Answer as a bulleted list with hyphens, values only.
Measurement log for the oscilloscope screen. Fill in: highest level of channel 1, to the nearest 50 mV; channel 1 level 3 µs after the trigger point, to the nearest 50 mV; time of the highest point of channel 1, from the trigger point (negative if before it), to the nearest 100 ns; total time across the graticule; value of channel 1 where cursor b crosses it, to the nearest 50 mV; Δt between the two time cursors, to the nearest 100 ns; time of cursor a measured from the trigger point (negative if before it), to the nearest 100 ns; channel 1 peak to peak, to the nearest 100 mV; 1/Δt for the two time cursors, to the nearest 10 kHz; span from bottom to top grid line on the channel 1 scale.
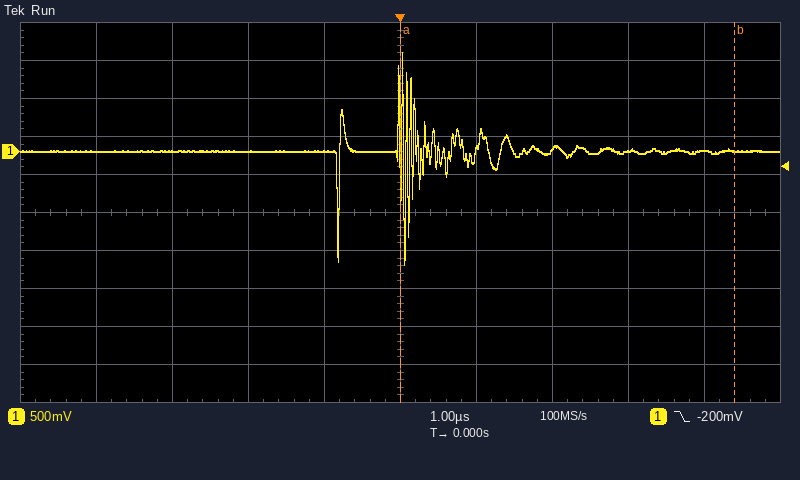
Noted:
- 1.30 V
- 0 mV
- 0.0 µs
- 10 µs
- 0 mV
- 4.4 µs
- 0.0 µs
- 2.80 V
- 230 kHz
- 5 V
